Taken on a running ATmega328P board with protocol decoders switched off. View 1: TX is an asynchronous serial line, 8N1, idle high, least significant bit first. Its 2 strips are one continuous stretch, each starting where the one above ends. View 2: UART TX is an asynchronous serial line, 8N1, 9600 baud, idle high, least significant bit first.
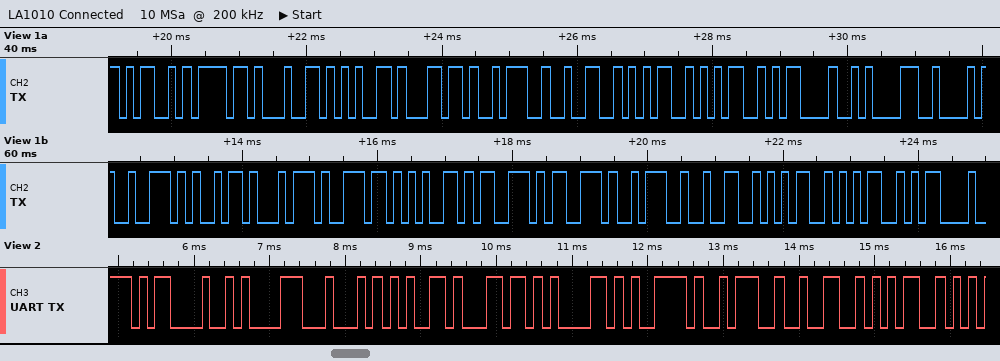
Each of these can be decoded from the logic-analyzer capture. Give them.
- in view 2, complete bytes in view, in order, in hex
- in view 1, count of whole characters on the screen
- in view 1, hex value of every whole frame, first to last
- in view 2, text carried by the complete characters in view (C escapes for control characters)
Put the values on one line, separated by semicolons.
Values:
0D 0A 44 65 6C 61 79 3A 32 35; 24; 4D 6F 64 65 6C 3A 32 35 35 0D 0A 42 72 69 74 6E 65 73 73 3A 32 35 35 0D; "\r\nDelay:25"
